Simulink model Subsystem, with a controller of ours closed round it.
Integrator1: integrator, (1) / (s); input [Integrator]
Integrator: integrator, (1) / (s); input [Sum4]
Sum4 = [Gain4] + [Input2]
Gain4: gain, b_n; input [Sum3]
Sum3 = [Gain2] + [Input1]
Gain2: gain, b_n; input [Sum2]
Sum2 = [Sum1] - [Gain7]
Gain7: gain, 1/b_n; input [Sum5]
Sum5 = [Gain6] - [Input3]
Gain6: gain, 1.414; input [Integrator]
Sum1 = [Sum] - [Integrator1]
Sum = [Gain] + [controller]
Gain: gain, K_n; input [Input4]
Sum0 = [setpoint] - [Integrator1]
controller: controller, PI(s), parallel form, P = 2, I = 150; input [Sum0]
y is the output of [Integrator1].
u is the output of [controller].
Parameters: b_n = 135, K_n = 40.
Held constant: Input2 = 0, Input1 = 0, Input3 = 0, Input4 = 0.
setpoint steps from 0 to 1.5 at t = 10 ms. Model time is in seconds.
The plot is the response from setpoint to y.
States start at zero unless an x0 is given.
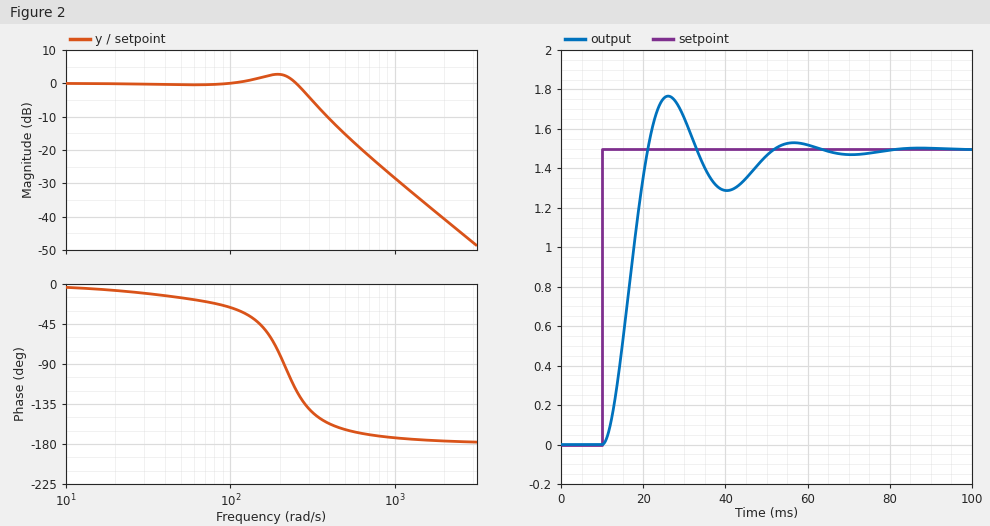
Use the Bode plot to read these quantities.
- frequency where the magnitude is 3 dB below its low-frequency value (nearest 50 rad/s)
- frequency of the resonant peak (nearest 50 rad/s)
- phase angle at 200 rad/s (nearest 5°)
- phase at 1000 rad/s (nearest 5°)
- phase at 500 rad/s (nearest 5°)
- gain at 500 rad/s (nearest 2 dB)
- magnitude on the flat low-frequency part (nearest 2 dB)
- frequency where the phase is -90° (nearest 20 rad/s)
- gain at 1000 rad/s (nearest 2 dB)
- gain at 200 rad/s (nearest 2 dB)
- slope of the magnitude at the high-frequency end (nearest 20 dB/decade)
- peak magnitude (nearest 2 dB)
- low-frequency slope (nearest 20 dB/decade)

300 rad/s
200 rad/s
-80°
-175°
-165°
-16 dB
0 dB
220 rad/s
-28 dB
2 dB
-40 dB/decade
2 dB
0 dB/decade
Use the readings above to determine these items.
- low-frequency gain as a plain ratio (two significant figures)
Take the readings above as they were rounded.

1.0
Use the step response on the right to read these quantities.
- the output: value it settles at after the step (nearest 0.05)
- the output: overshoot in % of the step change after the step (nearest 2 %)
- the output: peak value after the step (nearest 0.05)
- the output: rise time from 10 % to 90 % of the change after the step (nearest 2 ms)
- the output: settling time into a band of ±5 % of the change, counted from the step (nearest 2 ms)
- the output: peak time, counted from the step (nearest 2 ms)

1.50
18 %
1.75
8 ms
38 ms
16 ms
